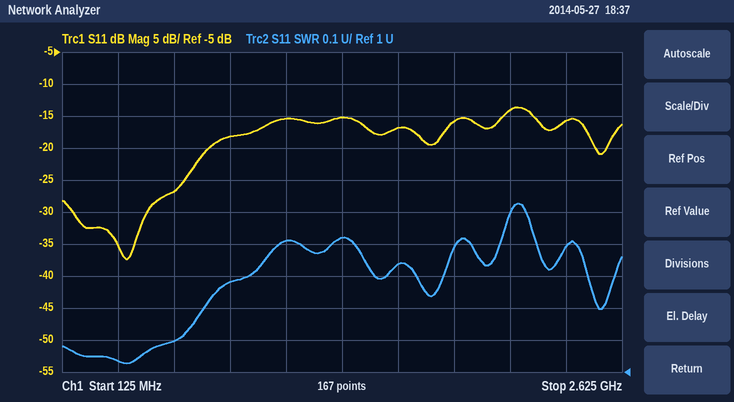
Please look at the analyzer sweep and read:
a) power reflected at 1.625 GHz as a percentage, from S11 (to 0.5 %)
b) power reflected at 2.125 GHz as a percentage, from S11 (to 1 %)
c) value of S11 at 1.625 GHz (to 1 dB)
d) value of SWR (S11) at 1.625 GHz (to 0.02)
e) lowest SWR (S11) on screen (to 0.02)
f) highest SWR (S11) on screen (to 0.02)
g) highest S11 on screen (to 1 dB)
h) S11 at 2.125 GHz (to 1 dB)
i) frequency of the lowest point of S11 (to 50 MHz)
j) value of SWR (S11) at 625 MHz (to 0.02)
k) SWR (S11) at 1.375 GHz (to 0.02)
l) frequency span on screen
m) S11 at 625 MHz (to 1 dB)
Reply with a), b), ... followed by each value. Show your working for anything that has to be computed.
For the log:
a) 10^(-17/10) ≈ 2.0 %
b) 10^(-14/10) ≈ 4 %
c) -17 dB
d) 1.34
e) 1.02
f) 1.52
g) -14 dB
h) -14 dB
i) 400 MHz
j) 1.10
k) 1.42
l) 2.5 GHz
m) -27 dB
